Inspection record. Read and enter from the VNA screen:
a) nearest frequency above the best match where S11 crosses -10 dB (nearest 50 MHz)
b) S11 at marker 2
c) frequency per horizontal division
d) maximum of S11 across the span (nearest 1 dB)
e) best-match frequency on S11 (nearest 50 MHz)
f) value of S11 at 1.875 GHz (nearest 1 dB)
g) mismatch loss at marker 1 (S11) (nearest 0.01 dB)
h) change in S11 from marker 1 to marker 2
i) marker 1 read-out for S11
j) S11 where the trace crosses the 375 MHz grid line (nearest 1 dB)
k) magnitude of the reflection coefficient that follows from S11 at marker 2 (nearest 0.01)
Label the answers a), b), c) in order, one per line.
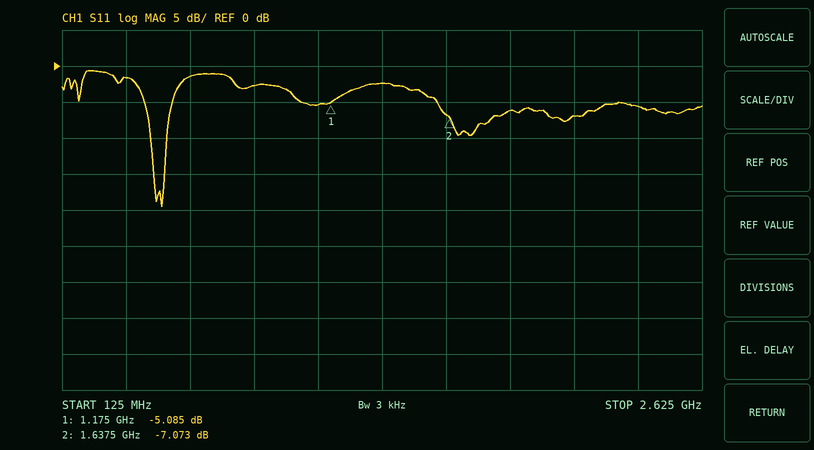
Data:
a) 550 MHz
b) -7.073 dB
c) 250 MHz
d) -1 dB
e) 500 MHz
f) -6 dB
g) 1.61 dB
h) -1.988 dB
i) -5.085 dB
j) -2 dB
k) 0.44
